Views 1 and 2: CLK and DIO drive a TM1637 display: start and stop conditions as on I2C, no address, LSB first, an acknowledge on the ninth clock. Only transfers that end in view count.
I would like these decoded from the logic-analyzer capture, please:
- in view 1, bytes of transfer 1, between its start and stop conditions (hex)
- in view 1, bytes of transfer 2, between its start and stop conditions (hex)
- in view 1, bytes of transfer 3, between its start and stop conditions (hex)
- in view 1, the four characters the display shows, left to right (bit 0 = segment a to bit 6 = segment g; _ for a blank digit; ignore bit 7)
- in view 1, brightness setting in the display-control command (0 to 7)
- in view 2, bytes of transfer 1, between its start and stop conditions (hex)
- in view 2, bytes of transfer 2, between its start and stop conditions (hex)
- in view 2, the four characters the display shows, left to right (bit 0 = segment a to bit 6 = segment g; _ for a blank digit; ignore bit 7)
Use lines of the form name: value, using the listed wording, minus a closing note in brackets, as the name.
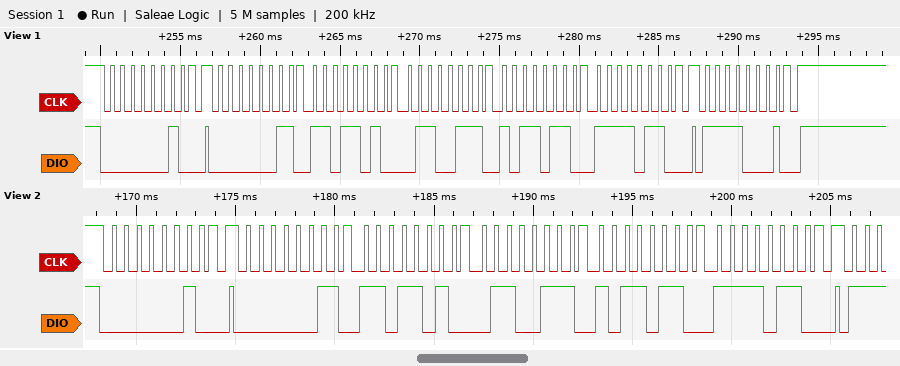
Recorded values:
in view 1, bytes of transfer 1, between its start and stop conditions: 40
in view 1, bytes of transfer 2, between its start and stop conditions: C0 5B E6 6D 6F
in view 1, bytes of transfer 3, between its start and stop conditions: 8F
in view 1, the four characters the display shows, left to right: 2459
in view 1, brightness setting in the display-control command: 7
in view 2, bytes of transfer 1, between its start and stop conditions: 40
in view 2, bytes of transfer 2, between its start and stop conditions: C0 5B E6 6D 6F
in view 2, the four characters the display shows, left to right: 2459
